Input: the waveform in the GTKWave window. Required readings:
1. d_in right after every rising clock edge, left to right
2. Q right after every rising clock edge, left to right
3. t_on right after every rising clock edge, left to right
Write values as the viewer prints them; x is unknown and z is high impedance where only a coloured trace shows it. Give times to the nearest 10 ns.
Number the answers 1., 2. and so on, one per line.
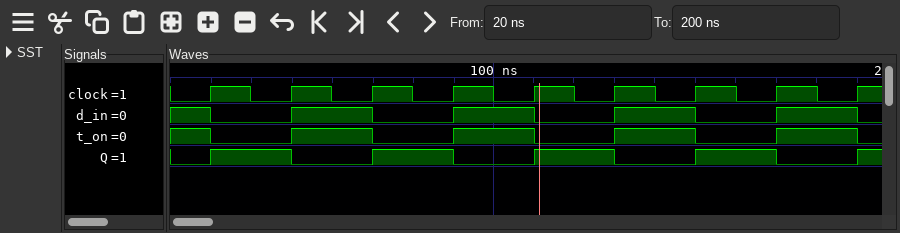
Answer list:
1. 0 1 0 1 0 1 0 1 0
2. 1 0 1 0 1 0 1 0 1
3. 0 1 0 1 0 1 0 1 0
